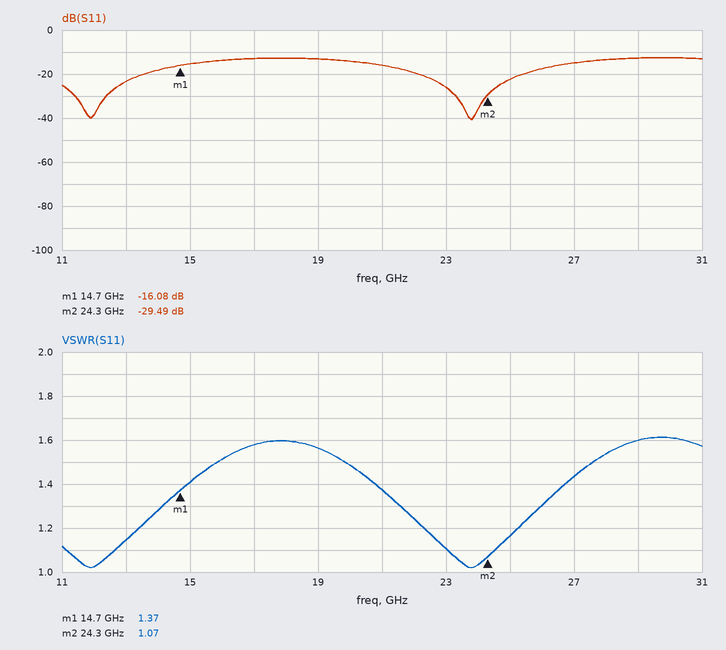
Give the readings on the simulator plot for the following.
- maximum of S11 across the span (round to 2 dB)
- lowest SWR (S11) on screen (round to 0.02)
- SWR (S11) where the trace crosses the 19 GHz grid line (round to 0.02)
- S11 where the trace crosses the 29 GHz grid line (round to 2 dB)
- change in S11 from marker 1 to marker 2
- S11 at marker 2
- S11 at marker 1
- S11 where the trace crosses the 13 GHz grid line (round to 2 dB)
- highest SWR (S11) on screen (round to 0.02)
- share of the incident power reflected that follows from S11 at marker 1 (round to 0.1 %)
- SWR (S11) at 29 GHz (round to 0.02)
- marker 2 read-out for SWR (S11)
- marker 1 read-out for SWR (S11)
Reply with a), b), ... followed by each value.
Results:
a) -12 dB
b) 1.02
c) 1.56
d) -12 dB
e) -13.41 dB
f) -29.49 dB
g) -16.08 dB
h) -24 dB
i) 1.62
j) 2.5 %
k) 1.60
l) 1.07
m) 1.37
